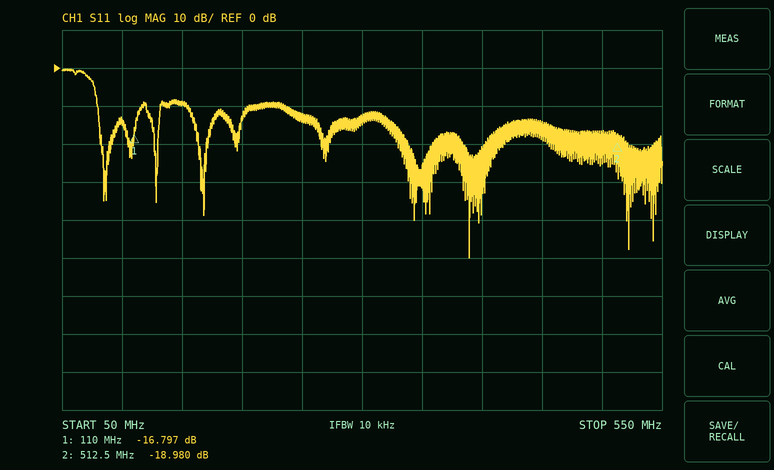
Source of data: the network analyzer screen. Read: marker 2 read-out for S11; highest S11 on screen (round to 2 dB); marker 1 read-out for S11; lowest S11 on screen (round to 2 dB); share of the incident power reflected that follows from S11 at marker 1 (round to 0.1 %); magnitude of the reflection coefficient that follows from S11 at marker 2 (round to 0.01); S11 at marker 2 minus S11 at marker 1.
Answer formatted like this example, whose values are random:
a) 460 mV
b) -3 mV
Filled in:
a) -18.980 dB
b) 0 dB
c) -16.797 dB
d) -50 dB
e) 2.1 %
f) 0.11
g) -2.183 dB
